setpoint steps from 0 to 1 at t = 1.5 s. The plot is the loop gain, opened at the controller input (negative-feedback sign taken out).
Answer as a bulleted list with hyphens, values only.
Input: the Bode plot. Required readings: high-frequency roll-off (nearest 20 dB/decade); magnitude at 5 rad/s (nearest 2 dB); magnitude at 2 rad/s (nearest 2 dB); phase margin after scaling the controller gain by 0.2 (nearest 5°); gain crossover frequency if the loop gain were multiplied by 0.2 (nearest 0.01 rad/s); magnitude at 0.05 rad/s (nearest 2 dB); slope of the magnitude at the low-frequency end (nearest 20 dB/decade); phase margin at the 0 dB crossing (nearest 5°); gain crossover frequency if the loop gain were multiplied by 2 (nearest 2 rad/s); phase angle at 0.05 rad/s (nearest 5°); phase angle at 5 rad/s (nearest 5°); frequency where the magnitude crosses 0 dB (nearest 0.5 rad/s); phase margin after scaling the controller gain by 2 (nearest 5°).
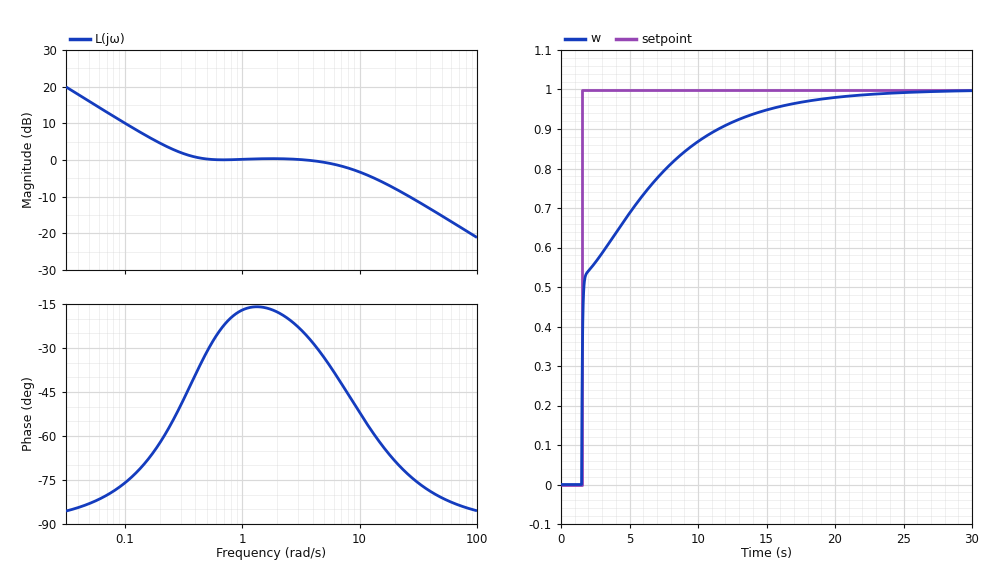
- -20 dB/decade
- 0 dB
- 0 dB
- 100°
- 0.06 rad/s
- 16 dB
- -20 dB/decade
- 155°
- 16 rad/s
- -85°
- -35°
- 3.5 rad/s
- 115°
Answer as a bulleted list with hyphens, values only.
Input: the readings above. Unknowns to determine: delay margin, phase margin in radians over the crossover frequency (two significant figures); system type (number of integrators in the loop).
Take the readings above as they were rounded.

- 0.77 s
- 1
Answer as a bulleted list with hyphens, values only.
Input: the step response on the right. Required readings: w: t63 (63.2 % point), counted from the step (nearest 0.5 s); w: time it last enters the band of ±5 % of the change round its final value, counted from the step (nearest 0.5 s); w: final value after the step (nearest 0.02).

- 2.5 s
- 13.5 s
- 1.00
